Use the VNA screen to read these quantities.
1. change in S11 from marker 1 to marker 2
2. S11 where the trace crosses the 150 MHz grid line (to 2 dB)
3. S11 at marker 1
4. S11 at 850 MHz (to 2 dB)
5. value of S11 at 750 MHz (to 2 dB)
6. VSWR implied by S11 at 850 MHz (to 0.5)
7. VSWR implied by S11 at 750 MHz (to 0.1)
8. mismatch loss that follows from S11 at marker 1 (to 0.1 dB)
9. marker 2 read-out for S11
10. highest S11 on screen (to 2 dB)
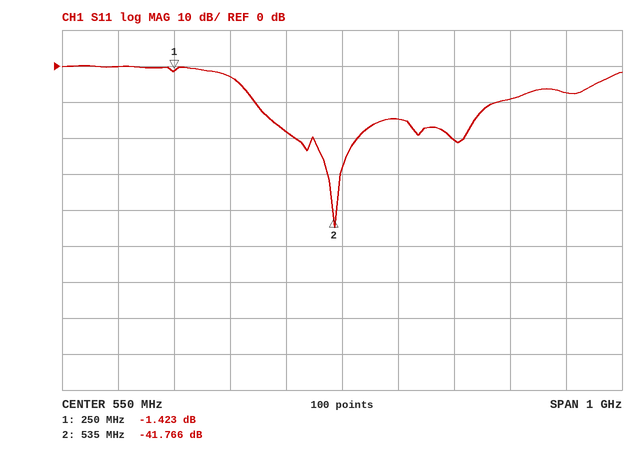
-40.343 dB
0 dB
-1.423 dB
-10 dB
-20 dB
2.0
1.2
5.5 dB
-41.766 dB
0 dB
